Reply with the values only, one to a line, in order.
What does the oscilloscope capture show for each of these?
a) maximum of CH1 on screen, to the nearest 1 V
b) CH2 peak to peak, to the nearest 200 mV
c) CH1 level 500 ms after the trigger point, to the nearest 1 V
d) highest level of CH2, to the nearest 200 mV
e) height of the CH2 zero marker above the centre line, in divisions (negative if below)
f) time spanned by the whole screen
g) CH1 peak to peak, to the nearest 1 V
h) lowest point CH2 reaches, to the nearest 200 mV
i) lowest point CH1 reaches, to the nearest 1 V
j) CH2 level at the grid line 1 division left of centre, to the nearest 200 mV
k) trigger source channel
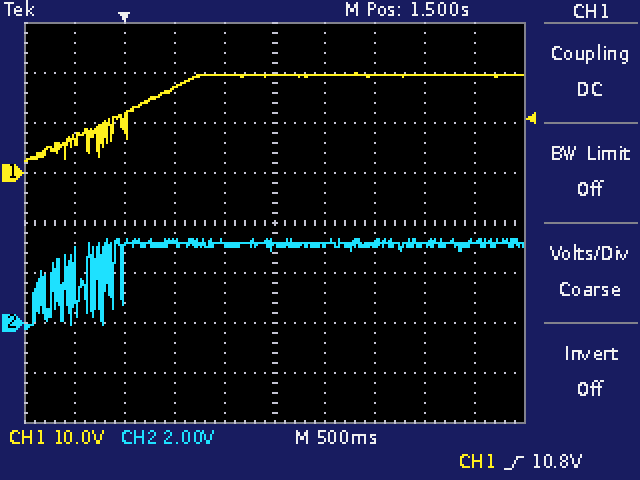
20 V
3.6 V
17 V
3.4 V
-2.0 div
5 s
18 V
-200 mV
2 V
3.2 V
CH1
